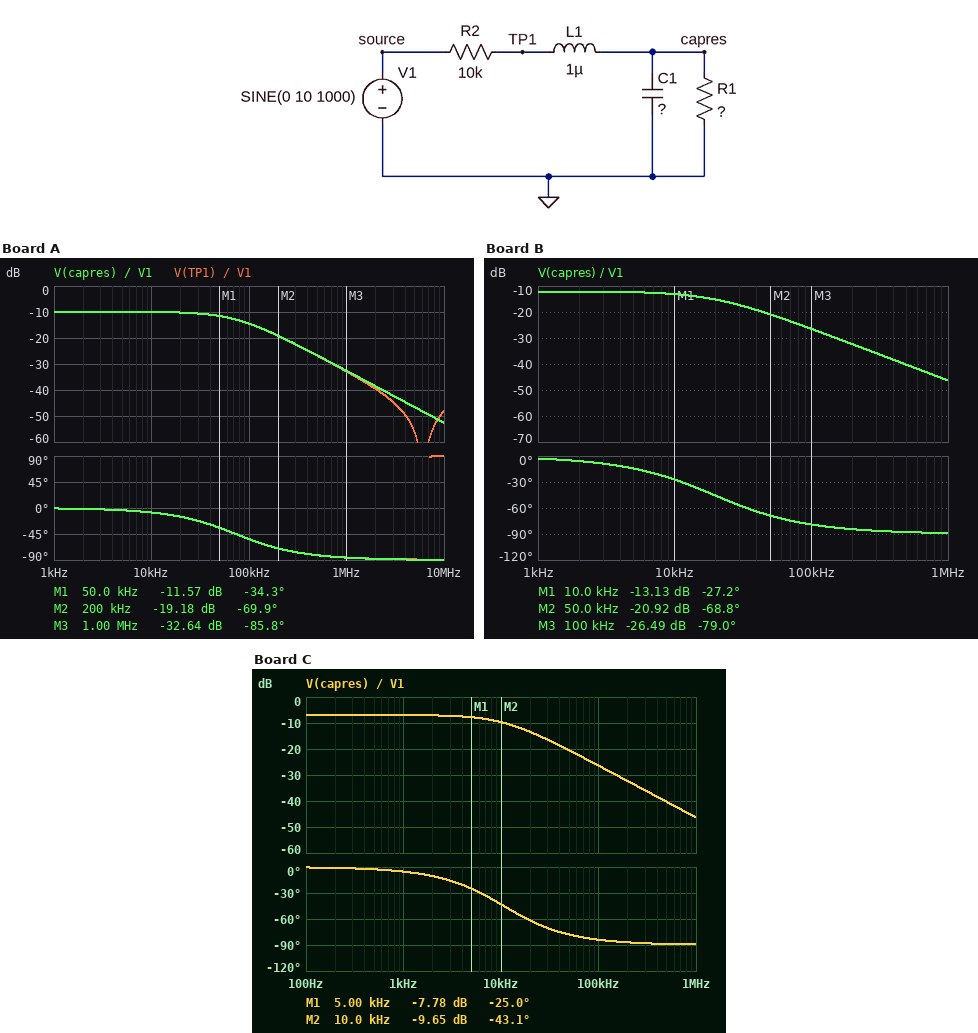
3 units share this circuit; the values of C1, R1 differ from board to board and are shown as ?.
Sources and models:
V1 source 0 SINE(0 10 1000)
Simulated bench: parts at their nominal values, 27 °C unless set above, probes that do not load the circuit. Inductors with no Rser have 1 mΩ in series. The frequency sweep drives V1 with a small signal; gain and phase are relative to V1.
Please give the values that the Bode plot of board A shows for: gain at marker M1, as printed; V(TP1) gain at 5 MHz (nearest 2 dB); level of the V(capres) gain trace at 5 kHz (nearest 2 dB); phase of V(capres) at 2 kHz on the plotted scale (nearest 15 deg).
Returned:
-11.57 dB
-56 dB
-10 dB
0 deg
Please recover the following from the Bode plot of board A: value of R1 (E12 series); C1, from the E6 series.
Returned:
4.7 kΩ
680 pF
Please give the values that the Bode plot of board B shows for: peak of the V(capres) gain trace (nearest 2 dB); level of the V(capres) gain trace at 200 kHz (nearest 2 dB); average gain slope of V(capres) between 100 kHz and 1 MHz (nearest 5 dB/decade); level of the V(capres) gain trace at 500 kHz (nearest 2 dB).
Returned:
-12 dB
-32 dB
-20 dB/decade
-40 dB
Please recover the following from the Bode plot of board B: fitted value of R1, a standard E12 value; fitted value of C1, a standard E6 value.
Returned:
3.3 kΩ
3.3 nF
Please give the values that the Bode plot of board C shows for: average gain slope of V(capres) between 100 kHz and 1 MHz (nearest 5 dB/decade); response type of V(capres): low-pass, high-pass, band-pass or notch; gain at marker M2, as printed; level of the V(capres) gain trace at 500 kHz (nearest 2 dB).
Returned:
-20 dB/decade
low-pass
-9.65 dB
-40 dB
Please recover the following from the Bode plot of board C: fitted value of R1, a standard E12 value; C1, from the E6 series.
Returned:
8.2 kΩ
3.3 nF
